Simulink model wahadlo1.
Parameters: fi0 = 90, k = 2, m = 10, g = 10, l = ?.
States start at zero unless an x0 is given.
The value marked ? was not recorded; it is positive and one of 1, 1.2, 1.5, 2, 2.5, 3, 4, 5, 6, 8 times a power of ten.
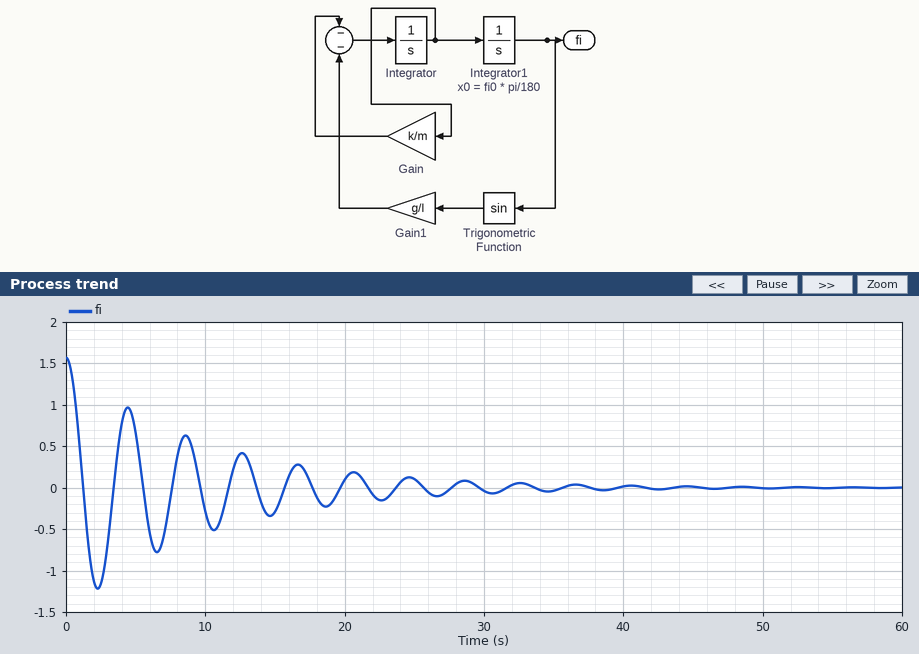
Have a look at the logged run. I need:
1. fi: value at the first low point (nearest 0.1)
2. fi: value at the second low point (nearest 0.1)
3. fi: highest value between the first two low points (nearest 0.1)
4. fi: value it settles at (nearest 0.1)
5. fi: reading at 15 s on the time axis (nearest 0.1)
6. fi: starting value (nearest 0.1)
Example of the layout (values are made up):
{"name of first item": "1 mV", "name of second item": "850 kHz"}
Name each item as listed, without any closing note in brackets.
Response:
{"fi: value at the first low point": "-1.2", "fi: value at the second low point": "-0.8", "fi: highest value between the first two low points": "1.0", "fi: value it settles at": "0.0", "fi: reading at 15 s on the time axis": "-0.3", "fi: starting value": "1.6"}
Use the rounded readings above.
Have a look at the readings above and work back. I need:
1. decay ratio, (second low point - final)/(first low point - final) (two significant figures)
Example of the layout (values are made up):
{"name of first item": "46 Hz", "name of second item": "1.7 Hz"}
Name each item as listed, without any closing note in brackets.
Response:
{"decay ratio, (second low point - final)/(first low point - final)": "0.67"}
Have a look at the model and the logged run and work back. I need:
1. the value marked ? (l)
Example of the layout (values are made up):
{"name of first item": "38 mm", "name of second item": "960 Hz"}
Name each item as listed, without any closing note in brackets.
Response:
{"the value marked ?": "4"}
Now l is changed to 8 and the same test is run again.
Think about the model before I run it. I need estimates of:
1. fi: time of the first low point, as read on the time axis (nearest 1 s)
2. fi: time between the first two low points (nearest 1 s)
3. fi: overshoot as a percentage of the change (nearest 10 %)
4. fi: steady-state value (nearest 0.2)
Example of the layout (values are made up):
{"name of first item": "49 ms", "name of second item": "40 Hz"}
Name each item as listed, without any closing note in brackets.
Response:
{"fi: time of the first low point, as read on the time axis": "3 s", "fi: time between the first two low points": "6 s", "fi: overshoot as a percentage of the change": "70 %", "fi: steady-state value": "0.0"}
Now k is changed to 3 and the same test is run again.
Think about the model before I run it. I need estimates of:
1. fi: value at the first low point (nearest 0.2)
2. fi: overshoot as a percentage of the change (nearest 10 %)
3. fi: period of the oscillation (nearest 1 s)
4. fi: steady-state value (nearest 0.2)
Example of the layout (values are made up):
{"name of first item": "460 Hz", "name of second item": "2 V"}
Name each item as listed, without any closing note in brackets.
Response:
{"fi: value at the first low point": "-1.0", "fi: overshoot as a percentage of the change": "70 %", "fi: period of the oscillation": "4 s", "fi: steady-state value": "0.0"}
